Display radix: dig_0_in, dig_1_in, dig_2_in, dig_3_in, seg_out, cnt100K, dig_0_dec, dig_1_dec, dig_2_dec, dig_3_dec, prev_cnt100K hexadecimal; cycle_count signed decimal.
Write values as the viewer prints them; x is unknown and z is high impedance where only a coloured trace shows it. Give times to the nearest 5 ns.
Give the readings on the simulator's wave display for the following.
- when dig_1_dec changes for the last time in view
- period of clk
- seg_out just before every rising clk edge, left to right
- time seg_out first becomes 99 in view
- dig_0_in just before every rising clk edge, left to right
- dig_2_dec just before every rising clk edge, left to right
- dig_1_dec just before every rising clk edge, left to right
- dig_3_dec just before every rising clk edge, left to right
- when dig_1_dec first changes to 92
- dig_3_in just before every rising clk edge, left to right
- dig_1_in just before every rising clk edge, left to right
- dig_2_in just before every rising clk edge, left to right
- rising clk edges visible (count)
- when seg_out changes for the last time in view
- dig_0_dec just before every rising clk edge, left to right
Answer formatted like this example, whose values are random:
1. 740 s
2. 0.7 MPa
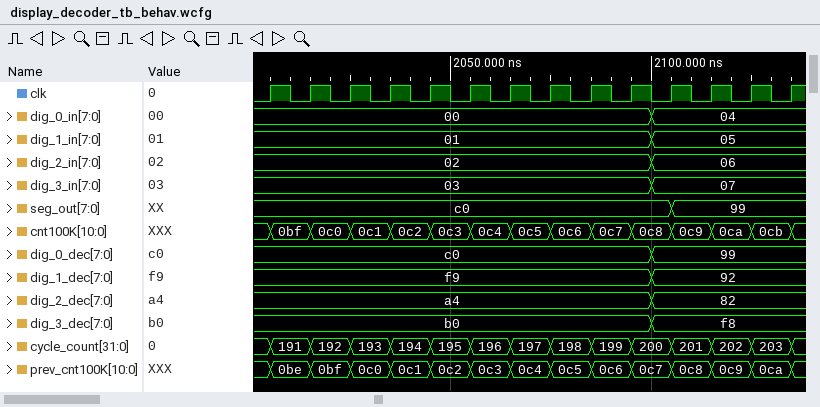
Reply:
1. 2100 ns
2. 10 ns
3. c0, c0, c0, c0, c0, c0, c0, c0, c0, c0, c0, 99, 99, 99
4. 2105 ns
5. 00, 00, 00, 00, 00, 00, 00, 00, 00, 00, 04, 04, 04, 04
6. a4, a4, a4, a4, a4, a4, a4, a4, a4, a4, 82, 82, 82, 82
7. f9, f9, f9, f9, f9, f9, f9, f9, f9, f9, 92, 92, 92, 92
8. b0, b0, b0, b0, b0, b0, b0, b0, b0, b0, f8, f8, f8, f8
9. 2100 ns
10. 03, 03, 03, 03, 03, 03, 03, 03, 03, 03, 07, 07, 07, 07
11. 01, 01, 01, 01, 01, 01, 01, 01, 01, 01, 05, 05, 05, 05
12. 02, 02, 02, 02, 02, 02, 02, 02, 02, 02, 06, 06, 06, 06
13. 14
14. 2105 ns
15. c0, c0, c0, c0, c0, c0, c0, c0, c0, c0, 99, 99, 99, 99
